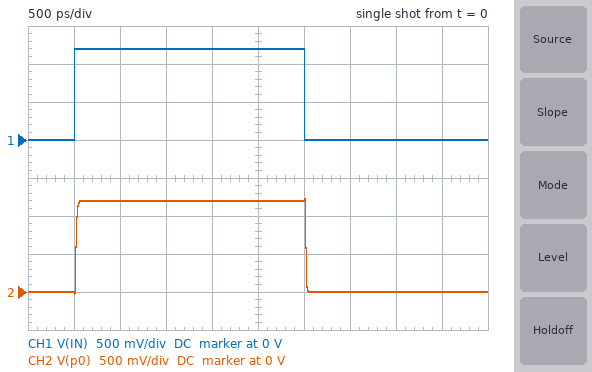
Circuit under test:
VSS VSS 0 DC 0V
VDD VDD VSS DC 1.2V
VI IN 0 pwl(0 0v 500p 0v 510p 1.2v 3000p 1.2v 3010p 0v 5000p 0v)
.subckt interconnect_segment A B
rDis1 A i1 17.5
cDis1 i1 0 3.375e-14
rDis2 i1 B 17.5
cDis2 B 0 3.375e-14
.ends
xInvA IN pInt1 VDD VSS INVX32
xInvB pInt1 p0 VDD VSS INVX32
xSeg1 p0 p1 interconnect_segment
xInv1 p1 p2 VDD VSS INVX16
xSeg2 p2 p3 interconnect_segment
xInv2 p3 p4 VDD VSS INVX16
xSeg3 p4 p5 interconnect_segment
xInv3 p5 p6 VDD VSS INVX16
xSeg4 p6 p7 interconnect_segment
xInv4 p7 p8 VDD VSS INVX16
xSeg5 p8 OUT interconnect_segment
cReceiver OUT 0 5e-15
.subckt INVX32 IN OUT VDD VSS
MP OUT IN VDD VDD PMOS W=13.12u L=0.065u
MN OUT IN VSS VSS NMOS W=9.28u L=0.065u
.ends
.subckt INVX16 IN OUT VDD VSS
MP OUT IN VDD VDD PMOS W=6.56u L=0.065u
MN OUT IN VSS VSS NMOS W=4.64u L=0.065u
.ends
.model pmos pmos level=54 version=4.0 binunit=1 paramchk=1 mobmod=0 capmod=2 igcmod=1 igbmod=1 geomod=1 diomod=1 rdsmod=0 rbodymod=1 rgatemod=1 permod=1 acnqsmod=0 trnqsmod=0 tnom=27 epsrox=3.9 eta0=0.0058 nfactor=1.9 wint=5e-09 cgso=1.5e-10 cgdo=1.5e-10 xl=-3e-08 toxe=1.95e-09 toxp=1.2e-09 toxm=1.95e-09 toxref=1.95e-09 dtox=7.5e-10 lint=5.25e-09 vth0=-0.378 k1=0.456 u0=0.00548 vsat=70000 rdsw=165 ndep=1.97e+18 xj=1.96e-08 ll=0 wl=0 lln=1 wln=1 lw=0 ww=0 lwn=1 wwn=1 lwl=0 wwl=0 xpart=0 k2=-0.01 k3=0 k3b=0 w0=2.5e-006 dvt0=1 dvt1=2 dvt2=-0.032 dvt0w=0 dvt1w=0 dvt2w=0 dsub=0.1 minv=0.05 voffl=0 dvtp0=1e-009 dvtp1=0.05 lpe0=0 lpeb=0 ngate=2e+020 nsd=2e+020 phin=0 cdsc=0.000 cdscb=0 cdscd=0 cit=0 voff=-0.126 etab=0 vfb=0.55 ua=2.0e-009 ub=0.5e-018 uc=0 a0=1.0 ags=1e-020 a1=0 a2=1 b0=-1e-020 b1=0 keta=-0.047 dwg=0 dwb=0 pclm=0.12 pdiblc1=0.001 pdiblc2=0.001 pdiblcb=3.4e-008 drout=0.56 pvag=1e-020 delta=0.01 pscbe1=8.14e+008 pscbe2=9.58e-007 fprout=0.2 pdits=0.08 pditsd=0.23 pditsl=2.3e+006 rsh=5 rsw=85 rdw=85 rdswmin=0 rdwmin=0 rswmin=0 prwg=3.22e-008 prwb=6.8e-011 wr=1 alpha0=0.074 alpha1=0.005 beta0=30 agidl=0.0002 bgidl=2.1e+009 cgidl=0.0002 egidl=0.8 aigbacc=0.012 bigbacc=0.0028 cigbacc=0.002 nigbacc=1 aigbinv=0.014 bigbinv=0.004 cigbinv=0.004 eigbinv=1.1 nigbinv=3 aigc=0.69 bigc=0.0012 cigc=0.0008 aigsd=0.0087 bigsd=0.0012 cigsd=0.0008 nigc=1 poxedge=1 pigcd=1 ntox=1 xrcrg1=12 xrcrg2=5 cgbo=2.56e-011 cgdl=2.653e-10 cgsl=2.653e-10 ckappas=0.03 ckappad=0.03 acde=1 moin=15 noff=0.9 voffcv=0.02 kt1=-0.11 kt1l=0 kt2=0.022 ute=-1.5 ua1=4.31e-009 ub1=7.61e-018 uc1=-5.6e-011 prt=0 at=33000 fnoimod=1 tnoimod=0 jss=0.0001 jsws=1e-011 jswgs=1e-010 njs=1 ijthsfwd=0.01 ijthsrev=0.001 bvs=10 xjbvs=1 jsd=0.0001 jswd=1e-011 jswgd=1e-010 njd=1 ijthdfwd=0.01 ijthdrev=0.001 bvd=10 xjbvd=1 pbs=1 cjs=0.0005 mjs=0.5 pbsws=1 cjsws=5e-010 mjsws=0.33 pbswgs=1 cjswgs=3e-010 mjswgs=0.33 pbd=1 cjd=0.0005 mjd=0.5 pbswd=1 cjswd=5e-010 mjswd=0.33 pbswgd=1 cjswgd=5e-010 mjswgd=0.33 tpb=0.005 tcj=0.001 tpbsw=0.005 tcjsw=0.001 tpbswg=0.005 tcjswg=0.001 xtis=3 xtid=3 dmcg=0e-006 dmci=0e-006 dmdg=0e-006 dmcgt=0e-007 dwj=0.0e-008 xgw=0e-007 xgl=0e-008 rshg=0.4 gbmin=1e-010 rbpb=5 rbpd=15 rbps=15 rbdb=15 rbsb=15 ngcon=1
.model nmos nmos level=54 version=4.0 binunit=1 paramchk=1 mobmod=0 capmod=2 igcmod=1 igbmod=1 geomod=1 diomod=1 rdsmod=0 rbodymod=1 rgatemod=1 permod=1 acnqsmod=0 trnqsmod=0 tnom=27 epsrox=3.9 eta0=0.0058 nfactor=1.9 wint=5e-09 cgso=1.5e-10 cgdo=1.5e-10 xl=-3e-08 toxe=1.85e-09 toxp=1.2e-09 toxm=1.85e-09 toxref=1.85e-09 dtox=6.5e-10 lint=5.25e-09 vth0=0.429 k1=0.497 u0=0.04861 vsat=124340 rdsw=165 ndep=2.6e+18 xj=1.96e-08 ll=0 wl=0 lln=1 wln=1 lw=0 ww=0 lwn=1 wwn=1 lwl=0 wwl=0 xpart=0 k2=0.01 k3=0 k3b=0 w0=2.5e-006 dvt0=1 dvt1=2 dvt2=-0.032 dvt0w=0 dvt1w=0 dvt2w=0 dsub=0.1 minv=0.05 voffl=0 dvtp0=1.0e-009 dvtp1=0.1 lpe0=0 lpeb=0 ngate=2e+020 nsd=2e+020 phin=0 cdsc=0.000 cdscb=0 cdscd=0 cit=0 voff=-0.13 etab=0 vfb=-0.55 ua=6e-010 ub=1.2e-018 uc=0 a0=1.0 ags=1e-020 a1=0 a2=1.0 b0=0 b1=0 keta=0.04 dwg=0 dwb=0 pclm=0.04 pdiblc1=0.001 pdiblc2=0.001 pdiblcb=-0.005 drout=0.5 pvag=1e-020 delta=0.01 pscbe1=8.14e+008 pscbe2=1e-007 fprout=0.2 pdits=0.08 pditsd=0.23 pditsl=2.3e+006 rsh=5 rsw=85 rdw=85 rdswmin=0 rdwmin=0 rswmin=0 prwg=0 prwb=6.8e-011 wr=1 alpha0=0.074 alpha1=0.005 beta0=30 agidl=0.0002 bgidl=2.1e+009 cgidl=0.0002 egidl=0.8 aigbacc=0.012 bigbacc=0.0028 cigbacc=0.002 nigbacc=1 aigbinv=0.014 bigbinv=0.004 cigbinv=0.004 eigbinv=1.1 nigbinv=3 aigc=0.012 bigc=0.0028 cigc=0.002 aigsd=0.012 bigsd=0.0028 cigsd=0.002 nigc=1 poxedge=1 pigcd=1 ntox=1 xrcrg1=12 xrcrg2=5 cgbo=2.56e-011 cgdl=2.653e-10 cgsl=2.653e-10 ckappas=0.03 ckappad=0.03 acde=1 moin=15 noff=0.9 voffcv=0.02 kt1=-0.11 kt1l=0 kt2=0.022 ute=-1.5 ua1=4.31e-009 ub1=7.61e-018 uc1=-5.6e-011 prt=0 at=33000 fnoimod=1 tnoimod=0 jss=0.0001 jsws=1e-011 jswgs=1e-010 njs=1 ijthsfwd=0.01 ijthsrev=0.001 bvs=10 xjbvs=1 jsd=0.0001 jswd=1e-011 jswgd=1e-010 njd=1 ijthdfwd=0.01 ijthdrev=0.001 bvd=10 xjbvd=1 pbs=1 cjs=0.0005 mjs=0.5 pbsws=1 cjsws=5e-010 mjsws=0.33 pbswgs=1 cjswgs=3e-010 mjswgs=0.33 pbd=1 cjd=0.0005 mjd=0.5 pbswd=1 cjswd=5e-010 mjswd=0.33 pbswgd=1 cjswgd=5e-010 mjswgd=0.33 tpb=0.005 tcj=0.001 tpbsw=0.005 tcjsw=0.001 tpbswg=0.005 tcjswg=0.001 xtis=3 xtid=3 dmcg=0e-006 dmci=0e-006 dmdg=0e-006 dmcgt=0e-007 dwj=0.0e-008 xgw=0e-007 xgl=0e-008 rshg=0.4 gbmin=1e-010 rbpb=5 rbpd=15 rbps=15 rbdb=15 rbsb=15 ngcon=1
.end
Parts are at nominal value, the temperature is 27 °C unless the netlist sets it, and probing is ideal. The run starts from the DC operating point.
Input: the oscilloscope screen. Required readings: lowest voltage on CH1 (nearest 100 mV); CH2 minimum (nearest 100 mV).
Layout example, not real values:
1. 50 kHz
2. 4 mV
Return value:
1. 0 V
2. 0 V
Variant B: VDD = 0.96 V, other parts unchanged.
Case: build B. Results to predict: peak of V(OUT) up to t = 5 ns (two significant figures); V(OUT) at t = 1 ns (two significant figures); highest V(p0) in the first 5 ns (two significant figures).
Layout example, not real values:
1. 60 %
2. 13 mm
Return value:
1. 970 mV
2. 960 mV
3. 990 mV
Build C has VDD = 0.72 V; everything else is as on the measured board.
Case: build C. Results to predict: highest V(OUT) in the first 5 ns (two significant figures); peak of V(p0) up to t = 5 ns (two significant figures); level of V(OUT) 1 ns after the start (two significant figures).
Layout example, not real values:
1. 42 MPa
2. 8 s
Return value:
1. 730 mV
2. 750 mV
3. 720 mV
